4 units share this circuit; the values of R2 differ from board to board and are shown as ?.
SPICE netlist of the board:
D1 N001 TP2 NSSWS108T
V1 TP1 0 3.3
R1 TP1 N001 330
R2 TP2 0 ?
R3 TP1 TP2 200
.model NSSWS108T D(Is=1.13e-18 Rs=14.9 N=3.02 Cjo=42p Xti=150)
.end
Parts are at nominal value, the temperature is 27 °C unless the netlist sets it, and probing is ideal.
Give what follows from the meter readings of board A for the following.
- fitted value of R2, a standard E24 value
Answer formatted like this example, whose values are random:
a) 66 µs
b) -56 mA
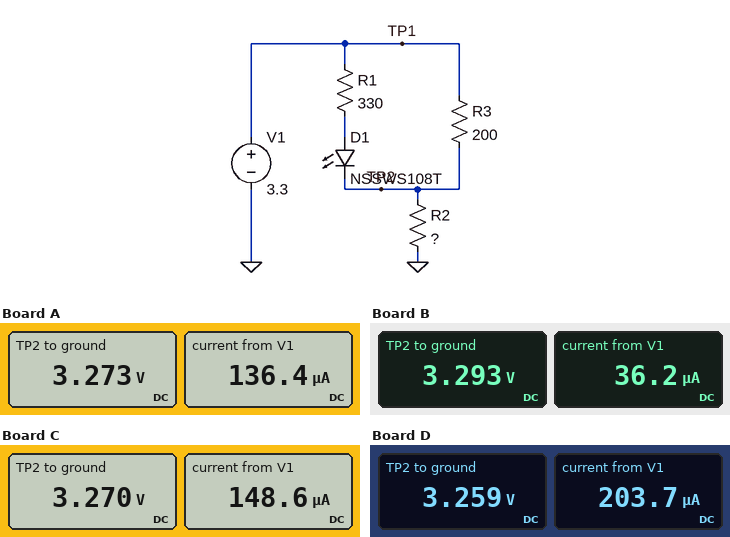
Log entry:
a) 24 kΩ
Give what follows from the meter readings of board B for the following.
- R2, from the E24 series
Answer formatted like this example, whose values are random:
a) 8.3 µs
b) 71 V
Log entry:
a) 91 kΩ
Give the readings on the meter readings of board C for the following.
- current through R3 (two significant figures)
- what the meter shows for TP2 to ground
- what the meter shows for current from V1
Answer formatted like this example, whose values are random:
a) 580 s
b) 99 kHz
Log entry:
a) 150 µA
b) 3.270 V
c) 148.6 µA
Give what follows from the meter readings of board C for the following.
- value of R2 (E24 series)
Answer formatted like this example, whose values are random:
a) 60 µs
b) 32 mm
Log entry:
a) 22 kΩ
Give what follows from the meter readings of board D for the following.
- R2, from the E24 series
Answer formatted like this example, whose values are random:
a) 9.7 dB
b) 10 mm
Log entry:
a) 16 kΩ
